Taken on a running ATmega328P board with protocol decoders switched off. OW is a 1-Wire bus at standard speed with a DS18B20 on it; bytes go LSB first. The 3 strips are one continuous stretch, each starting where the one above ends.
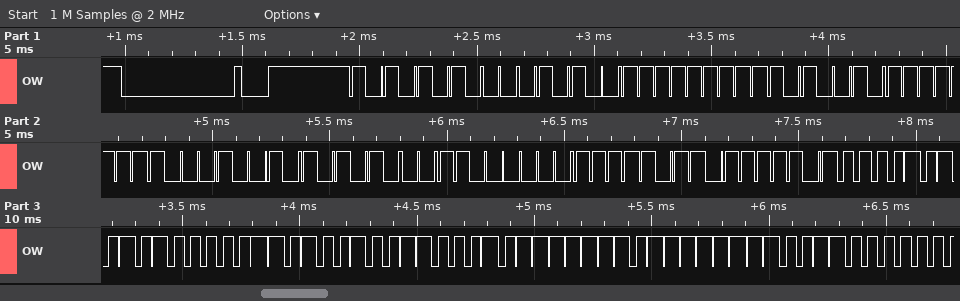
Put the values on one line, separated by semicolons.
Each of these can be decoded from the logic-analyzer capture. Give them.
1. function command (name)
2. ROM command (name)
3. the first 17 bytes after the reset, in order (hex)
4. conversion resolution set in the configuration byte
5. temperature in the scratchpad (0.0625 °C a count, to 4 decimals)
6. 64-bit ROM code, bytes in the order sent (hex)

Read Scratchpad; Match ROM; 55 28 FF 4B FF 48 15 03 DF BE 50 05 4B 46 7F FF 0C; 12 bits; 85.0000 °C; 28 FF 4B FF 48 15 03 DF
